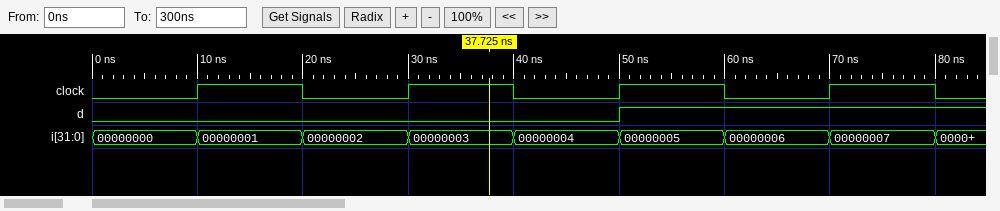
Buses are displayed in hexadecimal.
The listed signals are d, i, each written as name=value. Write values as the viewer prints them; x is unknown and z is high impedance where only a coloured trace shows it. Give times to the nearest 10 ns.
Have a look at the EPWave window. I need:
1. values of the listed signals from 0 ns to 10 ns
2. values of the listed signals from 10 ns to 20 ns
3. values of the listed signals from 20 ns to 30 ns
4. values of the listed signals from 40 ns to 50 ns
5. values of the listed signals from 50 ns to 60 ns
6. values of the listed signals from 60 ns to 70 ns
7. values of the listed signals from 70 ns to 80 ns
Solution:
d=0, i=00000000
d=0, i=00000001
d=0, i=00000002
d=0, i=00000004
d=1, i=00000005
d=1, i=00000006
d=1, i=00000007
